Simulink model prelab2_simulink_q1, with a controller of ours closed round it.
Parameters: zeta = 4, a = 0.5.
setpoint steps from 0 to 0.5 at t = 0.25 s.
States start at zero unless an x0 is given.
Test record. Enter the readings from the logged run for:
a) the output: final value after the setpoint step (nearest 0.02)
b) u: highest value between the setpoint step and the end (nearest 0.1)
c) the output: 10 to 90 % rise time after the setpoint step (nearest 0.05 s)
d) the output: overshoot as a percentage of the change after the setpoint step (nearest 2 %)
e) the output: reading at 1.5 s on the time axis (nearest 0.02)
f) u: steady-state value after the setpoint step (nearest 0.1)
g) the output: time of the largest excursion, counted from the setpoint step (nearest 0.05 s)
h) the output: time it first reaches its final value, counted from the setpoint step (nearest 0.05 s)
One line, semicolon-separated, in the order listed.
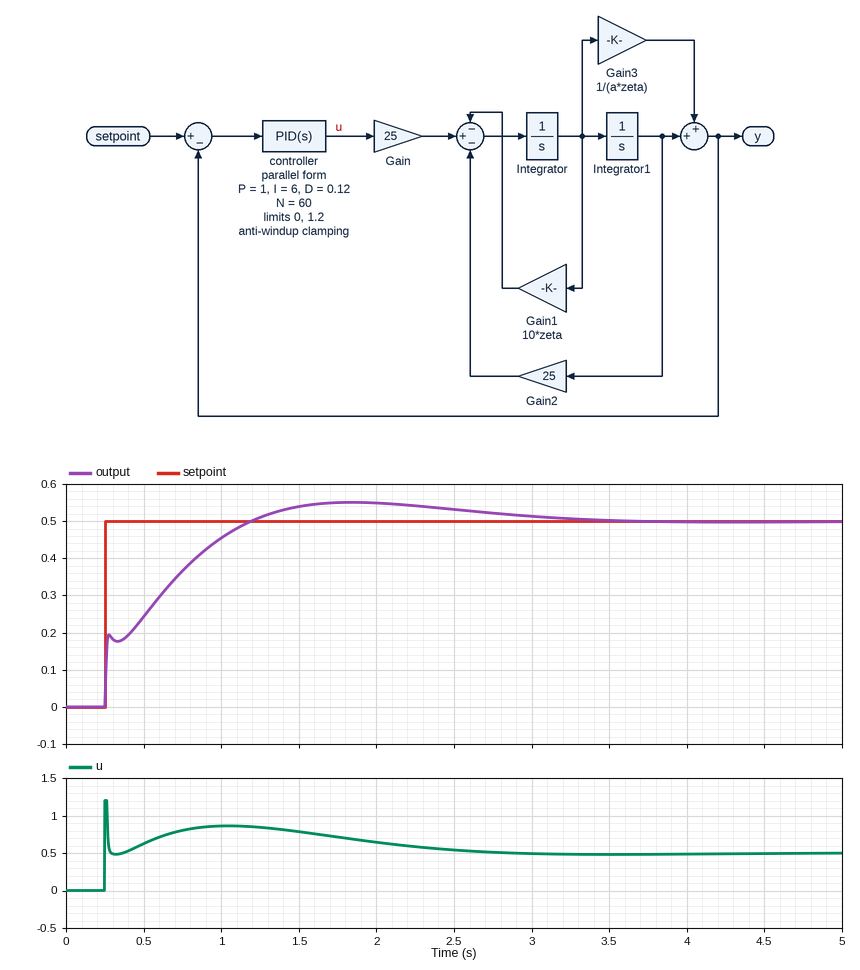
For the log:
0.50; 1.2; 0.75 s; 10 %; 0.54; 0.5; 1.60 s; 0.95 s
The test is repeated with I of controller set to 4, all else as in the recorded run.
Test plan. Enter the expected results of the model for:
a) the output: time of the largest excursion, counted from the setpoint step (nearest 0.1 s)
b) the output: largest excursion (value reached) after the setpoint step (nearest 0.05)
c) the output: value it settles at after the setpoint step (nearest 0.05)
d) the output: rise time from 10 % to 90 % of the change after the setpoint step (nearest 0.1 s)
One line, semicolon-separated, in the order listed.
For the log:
2.1 s; 0.55; 0.50; 1.0 s
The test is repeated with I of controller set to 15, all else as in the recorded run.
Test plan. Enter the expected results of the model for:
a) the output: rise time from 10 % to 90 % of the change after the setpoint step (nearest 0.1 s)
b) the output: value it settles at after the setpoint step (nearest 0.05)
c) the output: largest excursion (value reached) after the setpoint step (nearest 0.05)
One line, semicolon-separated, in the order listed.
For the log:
0.4 s; 0.50; 0.55
